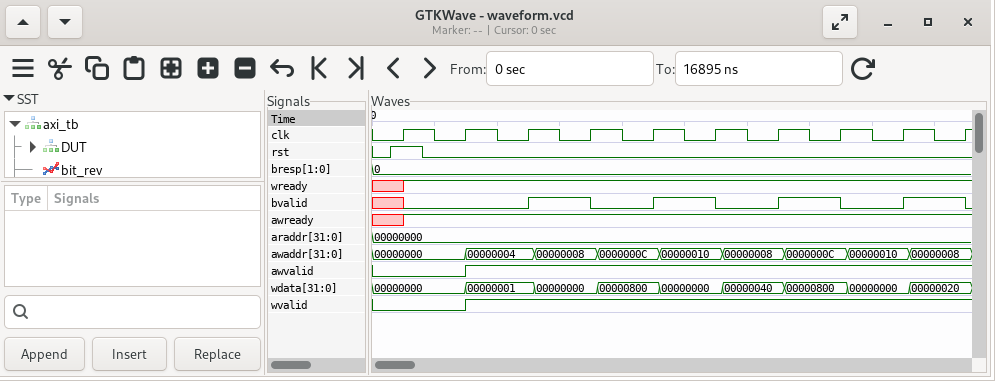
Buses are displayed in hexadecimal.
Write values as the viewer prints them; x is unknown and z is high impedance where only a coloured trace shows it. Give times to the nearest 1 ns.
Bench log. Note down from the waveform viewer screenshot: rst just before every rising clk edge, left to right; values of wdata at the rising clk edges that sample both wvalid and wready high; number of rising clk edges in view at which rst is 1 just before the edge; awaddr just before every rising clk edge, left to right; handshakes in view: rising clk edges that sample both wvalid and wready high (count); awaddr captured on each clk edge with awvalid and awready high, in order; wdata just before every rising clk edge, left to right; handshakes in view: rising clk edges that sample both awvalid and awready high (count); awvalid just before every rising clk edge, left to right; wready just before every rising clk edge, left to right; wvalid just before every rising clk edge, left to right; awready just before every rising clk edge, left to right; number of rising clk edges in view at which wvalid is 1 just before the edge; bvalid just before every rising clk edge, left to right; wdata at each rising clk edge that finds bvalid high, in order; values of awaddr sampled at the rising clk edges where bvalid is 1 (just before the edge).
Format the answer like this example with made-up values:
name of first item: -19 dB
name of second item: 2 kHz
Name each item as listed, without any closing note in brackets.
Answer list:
rst just before every rising clk edge, left to right: 1 0 0 0 0 0 0 0 0 0
values of wdata at the rising clk edges that sample both wvalid and wready high: 00000001, 00000000, 00000800, 00000000, 00000040, 00000800, 00000000, 00000020
number of rising clk edges in view at which rst is 1 just before the edge: 1
awaddr just before every rising clk edge, left to right: 00000000, 00000000, 00000004, 00000008, 0000000C, 00000010, 00000008, 0000000C, 00000010, 00000008
handshakes in view: rising clk edges that sample both wvalid and wready high: 8
awaddr captured on each clk edge with awvalid and awready high, in order: 00000004, 00000008, 0000000C, 00000010, 00000008, 0000000C, 00000010, 00000008
wdata just before every rising clk edge, left to right: 00000000, 00000000, 00000001, 00000000, 00000800, 00000000, 00000040, 00000800, 00000000, 00000020
handshakes in view: rising clk edges that sample both awvalid and awready high: 8
awvalid just before every rising clk edge, left to right: 0 0 1 1 1 1 1 1 1 1
wready just before every rising clk edge, left to right: x 1 1 1 1 1 1 1 1 1
wvalid just before every rising clk edge, left to right: 0 0 1 1 1 1 1 1 1 1
awready just before every rising clk edge, left to right: x 1 1 1 1 1 1 1 1 1
number of rising clk edges in view at which wvalid is 1 just before the edge: 8
bvalid just before every rising clk edge, left to right: x 0 0 1 0 1 0 1 0 1
wdata at each rising clk edge that finds bvalid high, in order: 00000000, 00000000, 00000800, 00000020
values of awaddr sampled at the rising clk edges where bvalid is 1: 00000008, 00000010, 0000000C, 00000008
